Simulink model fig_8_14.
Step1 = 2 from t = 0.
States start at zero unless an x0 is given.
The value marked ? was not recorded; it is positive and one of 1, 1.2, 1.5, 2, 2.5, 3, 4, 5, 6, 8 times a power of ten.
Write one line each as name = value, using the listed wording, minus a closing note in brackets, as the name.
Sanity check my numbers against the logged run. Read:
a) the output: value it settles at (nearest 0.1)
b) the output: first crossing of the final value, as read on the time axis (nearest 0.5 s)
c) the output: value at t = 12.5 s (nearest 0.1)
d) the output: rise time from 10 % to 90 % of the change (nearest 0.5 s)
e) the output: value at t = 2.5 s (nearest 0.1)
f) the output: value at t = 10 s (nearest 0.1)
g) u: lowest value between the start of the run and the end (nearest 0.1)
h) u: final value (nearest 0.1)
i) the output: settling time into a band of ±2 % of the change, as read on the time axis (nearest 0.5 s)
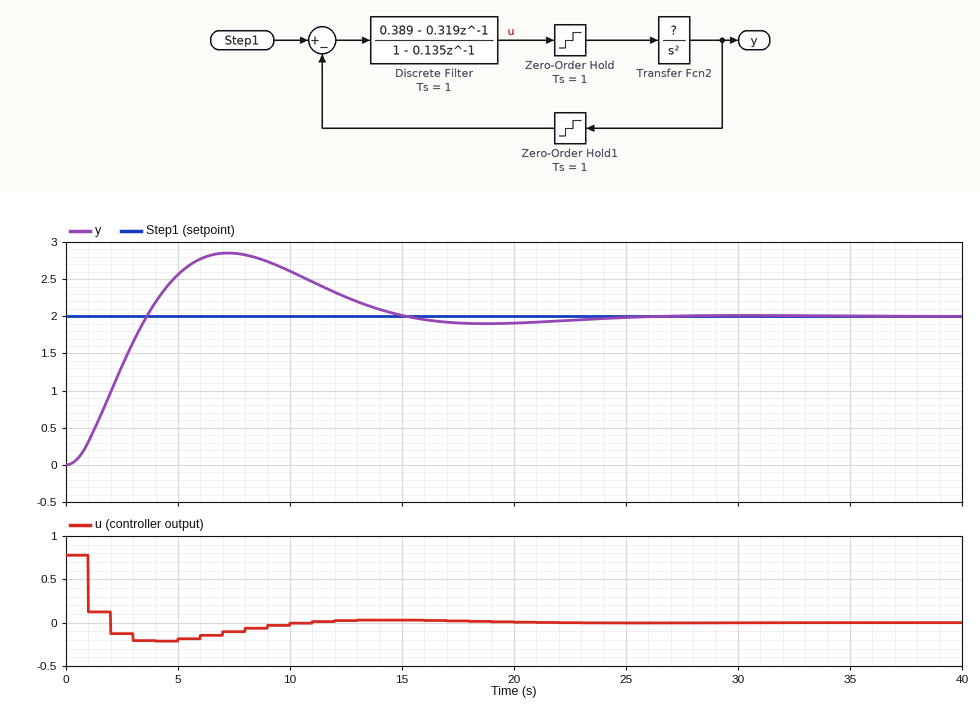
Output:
the output: value it settles at = 2.0
the output: first crossing of the final value, as read on the time axis = 3.5 s
the output: value at t = 12.5 s = 2.3
the output: rise time from 10 % to 90 % of the change = 2.5 s
the output: value at t = 2.5 s = 1.3
the output: value at t = 10 s = 2.6
u: lowest value between the start of the run and the end = -0.2
u: final value = 0.0
the output: settling time into a band of ±2 % of the change, as read on the time axis = 23.5 s
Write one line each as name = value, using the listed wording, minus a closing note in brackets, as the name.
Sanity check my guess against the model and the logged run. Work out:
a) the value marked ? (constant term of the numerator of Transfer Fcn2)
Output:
the value marked ? = 0.8
